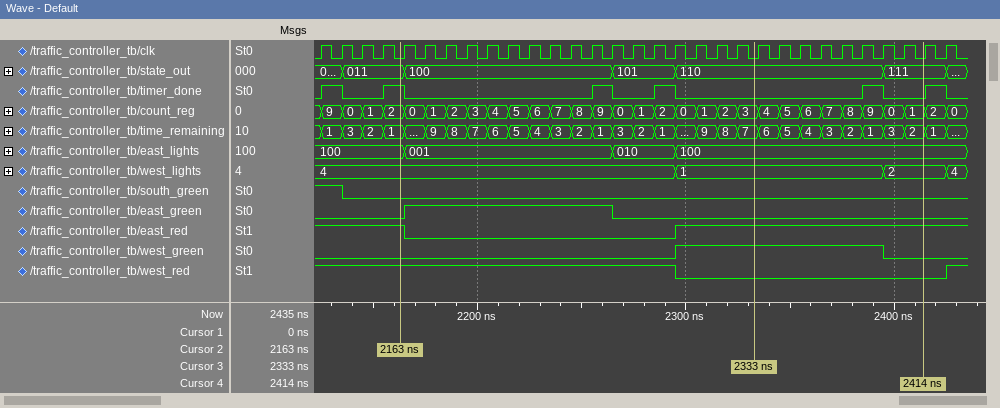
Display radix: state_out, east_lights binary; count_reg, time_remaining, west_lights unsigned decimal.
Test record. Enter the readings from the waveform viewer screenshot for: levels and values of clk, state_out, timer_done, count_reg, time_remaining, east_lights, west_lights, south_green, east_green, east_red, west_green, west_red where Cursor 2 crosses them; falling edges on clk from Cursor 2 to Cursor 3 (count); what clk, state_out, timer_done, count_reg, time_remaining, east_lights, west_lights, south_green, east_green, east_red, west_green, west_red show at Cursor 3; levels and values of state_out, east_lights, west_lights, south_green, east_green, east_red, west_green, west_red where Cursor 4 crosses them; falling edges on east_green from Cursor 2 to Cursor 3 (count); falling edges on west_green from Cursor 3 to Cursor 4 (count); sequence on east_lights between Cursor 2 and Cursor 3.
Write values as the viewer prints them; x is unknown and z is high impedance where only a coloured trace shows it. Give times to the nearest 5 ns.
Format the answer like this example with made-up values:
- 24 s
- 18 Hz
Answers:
- clk=0, state_out=011, timer_done=1, count_reg=2, time_remaining=1, east_lights=100, west_lights=4, south_green=0, east_green=0, east_red=1, west_green=0, west_red=1
- 17
- clk=0, state_out=110, timer_done=0, count_reg=3, time_remaining=7, east_lights=100, west_lights=1, south_green=0, east_green=0, east_red=1, west_green=1, west_red=0
- state_out=111, east_lights=100, west_lights=2, south_green=0, east_green=0, east_red=1, west_green=0, west_red=0
- 1
- 1
- 100, 001, 010, 100
